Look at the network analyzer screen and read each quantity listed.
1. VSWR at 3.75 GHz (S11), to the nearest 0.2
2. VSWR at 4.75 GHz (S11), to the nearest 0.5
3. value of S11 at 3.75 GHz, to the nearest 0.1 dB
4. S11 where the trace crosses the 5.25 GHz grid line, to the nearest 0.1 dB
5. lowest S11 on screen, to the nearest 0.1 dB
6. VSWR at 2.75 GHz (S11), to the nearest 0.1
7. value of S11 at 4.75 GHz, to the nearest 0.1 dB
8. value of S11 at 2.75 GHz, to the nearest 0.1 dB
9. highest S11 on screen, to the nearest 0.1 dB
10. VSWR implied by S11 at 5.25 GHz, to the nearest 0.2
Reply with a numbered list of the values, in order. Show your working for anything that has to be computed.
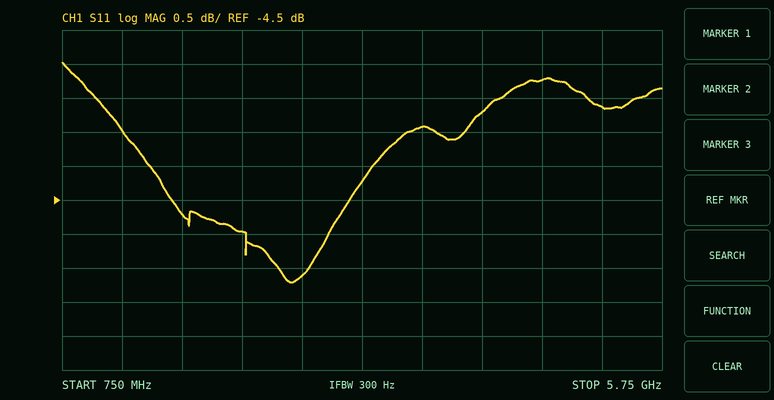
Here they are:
1. |Γ| = 10^(-3.4/20) = 0.6761; VSWR = (1 + 0.6761)/(1 − 0.6761) ≈ 5.2
2. |Γ| = 10^(-2.7/20) = 0.7328; VSWR = (1 + 0.7328)/(1 − 0.7328) ≈ 6.5
3. -3.4 dB
4. -3.1 dB
5. -5.7 dB
6. |Γ| = 10^(-5.6/20) = 0.5248; VSWR = (1 + 0.5248)/(1 − 0.5248) ≈ 3.2
7. -2.7 dB
8. -5.6 dB
9. -2.5 dB
10. |Γ| = 10^(-3.1/20) = 0.6998; VSWR = (1 + 0.6998)/(1 − 0.6998) ≈ 5.66, so 5.6 to the nearest 0.2
